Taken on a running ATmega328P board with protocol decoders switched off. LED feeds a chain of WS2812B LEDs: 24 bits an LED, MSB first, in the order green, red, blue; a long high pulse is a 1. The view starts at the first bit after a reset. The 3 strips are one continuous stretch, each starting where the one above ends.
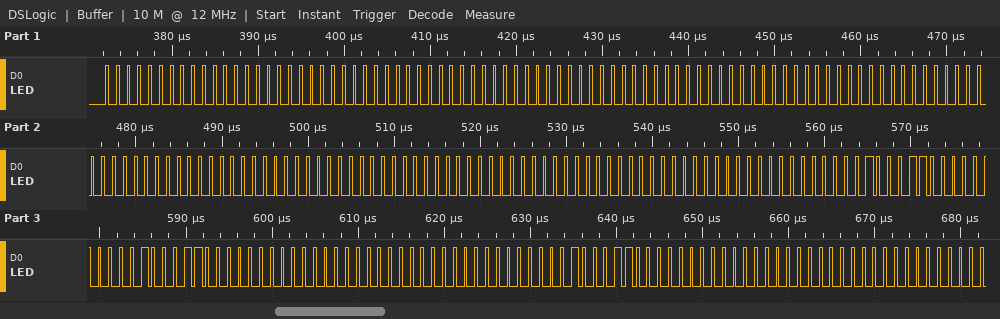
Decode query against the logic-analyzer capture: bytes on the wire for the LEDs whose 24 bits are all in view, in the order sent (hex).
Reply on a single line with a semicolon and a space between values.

00 00 00 00 00 00 00 00 00 00 00 00 00 00 00 00 00 00 00 23 00 23 00 00 00 00 23 00 00 00
